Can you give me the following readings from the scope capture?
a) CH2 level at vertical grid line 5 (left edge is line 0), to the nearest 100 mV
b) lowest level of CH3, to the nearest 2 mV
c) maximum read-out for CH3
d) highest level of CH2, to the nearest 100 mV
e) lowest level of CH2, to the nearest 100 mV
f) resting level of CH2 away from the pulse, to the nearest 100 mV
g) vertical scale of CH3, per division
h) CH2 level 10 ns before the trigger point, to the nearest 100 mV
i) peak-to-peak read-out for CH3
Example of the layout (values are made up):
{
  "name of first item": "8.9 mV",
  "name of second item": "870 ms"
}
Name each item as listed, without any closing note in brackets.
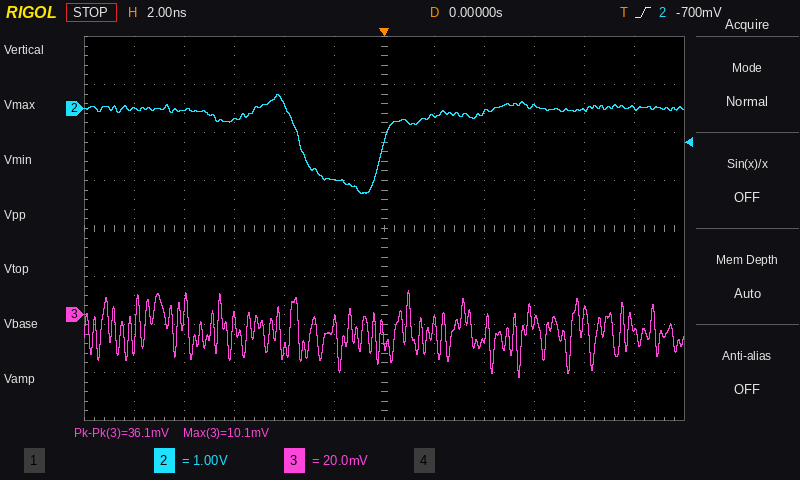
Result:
{
  "CH2 level at vertical grid line 5 (left edge is line 0), to the nearest 100 mV": "-1.5 V",
  "lowest level of CH3, to the nearest 2 mV": "-26 mV",
  "maximum read-out for CH3": "10.1 mV",
  "highest level of CH2, to the nearest 100 mV": "300 mV",
  "lowest level of CH2, to the nearest 100 mV": "-1.8 V",
  "resting level of CH2 away from the pulse, to the nearest 100 mV": "0.0 V",
  "vertical scale of CH3, per division": "20 mV",
  "CH2 level 10 ns before the trigger point, to the nearest 100 mV": "0.0 V",
  "peak-to-peak read-out for CH3": "36.1 mV"
}
